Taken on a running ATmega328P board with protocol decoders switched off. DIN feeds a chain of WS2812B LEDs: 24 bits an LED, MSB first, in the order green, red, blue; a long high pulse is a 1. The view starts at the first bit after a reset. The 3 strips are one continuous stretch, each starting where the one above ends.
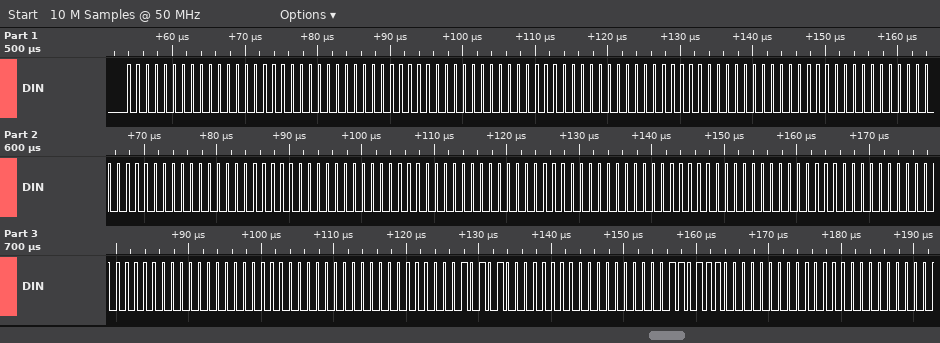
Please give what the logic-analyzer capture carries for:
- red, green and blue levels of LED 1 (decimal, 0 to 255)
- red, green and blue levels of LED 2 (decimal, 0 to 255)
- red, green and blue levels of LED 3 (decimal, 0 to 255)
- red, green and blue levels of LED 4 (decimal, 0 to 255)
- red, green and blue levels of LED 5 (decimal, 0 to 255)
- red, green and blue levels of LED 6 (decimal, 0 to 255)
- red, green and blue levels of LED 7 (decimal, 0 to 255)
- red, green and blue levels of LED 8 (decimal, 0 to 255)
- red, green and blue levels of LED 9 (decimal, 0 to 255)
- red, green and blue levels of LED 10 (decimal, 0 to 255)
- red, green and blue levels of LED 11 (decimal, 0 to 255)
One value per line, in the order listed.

0, 0, 0
0, 0, 0
0, 0, 0
0, 0, 0
0, 0, 0
0, 0, 0
0, 0, 0
0, 0, 0
0, 0, 0
0, 21, 0
0, 55, 0
